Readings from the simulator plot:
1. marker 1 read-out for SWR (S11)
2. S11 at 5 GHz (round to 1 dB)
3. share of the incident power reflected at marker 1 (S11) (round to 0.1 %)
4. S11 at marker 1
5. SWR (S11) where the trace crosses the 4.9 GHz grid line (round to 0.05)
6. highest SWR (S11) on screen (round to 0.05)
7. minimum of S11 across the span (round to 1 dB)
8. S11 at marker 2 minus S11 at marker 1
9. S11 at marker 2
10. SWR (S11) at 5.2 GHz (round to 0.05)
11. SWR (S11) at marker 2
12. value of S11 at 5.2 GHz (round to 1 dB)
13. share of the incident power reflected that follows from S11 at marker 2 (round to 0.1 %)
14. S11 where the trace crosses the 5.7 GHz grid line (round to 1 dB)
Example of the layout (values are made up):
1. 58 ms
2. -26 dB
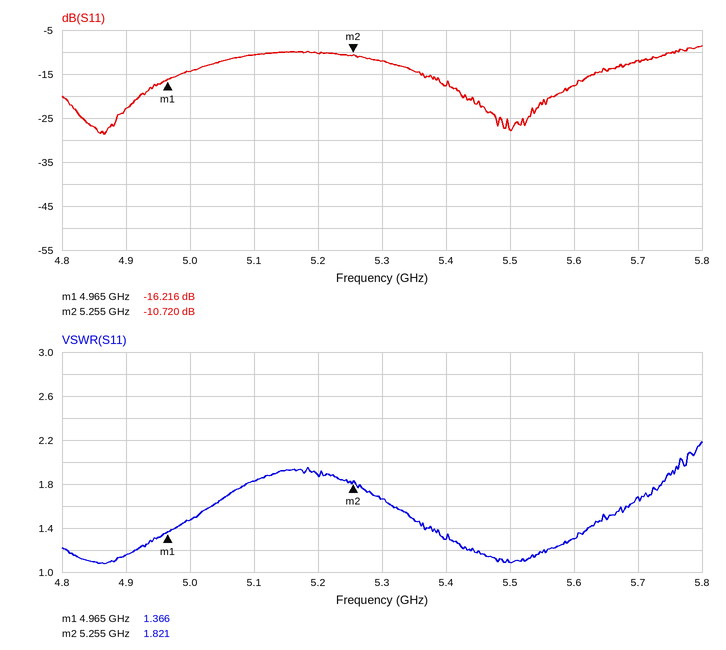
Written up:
1. 1.366
2. -14 dB
3. 2.4 %
4. -16.216 dB
5. 1.15
6. 2.20
7. -29 dB
8. 5.496 dB
9. -10.720 dB
10. 1.90
11. 1.821
12. -10 dB
13. 8.5 %
14. -12 dB
